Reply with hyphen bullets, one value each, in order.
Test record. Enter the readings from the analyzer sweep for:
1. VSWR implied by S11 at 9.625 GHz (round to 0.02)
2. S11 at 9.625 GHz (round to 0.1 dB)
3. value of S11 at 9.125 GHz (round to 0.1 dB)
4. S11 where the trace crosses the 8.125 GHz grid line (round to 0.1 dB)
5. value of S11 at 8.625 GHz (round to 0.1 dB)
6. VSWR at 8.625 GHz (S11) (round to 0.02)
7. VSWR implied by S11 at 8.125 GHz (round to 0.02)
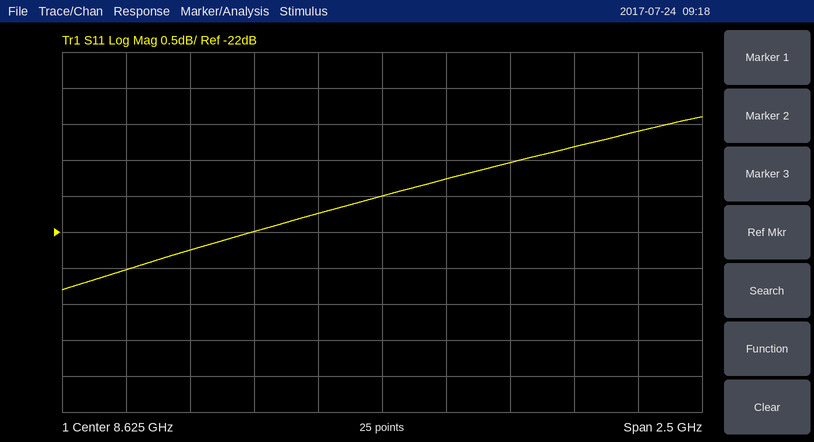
- 1.20
- -20.6 dB
- -21.0 dB
- -22.0 dB
- -21.5 dB
- 1.18
- 1.18
